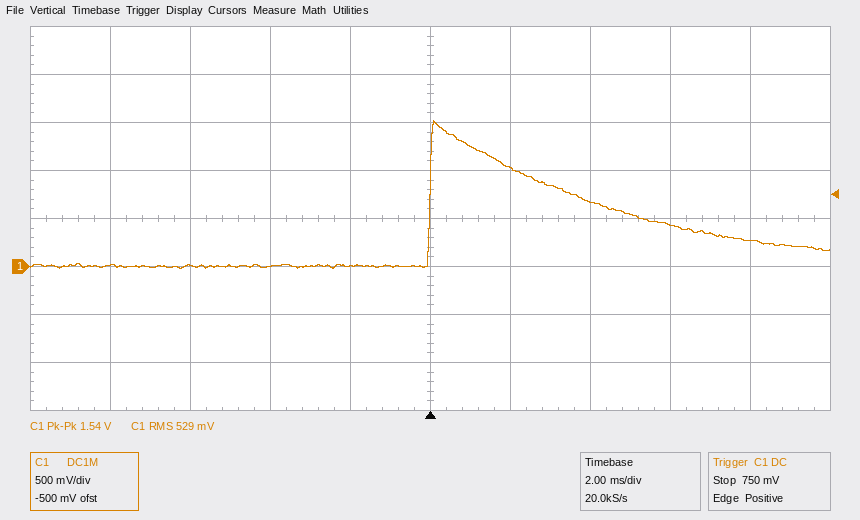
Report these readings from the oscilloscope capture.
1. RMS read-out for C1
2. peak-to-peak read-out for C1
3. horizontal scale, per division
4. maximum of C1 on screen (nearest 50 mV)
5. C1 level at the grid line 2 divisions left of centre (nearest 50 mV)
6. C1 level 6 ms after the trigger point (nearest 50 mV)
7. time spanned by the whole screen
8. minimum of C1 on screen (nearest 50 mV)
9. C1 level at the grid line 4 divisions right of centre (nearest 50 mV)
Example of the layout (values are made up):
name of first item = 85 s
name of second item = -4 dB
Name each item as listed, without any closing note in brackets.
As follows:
RMS read-out for C1 = 529 mV
peak-to-peak read-out for C1 = 1.54 V
horizontal scale, per division = 2 ms
maximum of C1 on screen = 1.50 V
C1 level at the grid line 2 divisions left of centre = 0 mV
C1 level 6 ms after the trigger point = 450 mV
time spanned by the whole screen = 20 ms
minimum of C1 on screen = 0 mV
C1 level at the grid line 4 divisions right of centre = 250 mV
